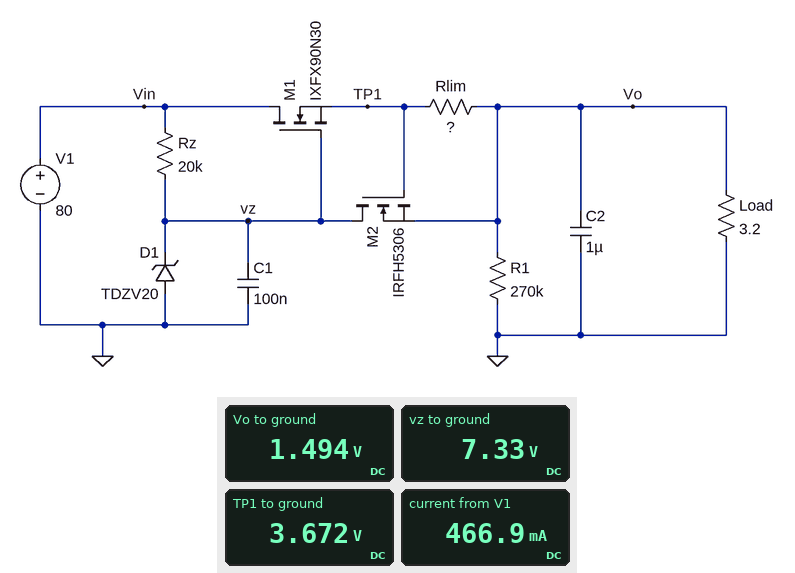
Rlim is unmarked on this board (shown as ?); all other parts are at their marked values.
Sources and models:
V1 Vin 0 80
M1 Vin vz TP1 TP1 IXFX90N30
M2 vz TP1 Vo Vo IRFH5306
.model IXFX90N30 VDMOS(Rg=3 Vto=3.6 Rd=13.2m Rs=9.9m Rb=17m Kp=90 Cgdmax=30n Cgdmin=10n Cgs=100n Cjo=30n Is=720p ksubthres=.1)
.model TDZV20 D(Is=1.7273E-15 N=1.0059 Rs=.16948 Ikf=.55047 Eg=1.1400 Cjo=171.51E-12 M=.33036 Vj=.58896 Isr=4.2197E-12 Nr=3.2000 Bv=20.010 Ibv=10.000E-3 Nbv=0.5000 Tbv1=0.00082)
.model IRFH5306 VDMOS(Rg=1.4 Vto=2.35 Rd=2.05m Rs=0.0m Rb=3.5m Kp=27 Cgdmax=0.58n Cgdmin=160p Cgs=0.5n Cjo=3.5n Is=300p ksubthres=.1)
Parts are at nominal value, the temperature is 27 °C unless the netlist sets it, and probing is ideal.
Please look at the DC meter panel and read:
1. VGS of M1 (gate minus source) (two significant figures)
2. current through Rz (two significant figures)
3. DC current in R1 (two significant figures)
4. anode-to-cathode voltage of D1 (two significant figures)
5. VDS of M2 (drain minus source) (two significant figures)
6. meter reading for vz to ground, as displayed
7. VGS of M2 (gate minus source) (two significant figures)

3.7 V
3.6 mA
5.5 µA
-7.3 V
5.8 V
7.33 V
2.2 V
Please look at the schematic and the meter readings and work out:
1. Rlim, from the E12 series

4.7 Ω
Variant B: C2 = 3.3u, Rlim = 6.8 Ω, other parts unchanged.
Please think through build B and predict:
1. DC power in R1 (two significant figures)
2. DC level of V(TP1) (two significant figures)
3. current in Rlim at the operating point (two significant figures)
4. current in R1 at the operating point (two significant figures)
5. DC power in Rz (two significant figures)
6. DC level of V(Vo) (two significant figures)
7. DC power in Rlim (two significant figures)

4.0 µW
3.2 V
320 mA
3.8 µA
270 mW
1.0 V
700 mW
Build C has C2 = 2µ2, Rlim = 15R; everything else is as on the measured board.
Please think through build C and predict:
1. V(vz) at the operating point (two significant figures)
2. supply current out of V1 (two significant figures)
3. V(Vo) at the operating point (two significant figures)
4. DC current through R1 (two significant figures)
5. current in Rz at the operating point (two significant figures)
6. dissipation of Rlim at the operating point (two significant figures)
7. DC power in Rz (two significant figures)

6.2 V
150 mA
480 mV
1.8 µA
3.7 mA
320 mW
270 mW
